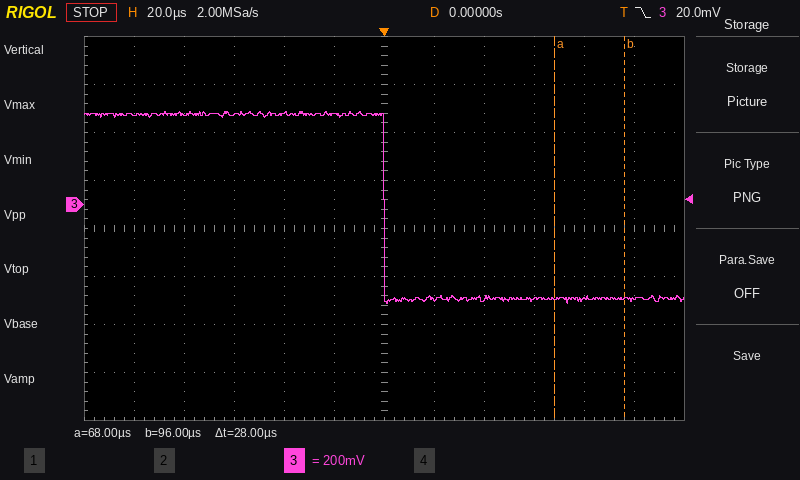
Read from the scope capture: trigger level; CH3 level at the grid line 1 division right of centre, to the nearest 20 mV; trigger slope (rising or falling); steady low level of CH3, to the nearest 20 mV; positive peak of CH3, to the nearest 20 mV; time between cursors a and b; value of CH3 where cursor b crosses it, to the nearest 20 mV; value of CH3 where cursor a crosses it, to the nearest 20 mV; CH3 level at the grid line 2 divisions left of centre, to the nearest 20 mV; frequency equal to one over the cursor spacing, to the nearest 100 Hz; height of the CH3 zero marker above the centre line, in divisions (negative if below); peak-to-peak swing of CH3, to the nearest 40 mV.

20.0 mV
-400 mV
falling
-400 mV
380 mV
28 µs
-400 mV
-400 mV
380 mV
35.7 kHz
+0.5 div
800 mV
